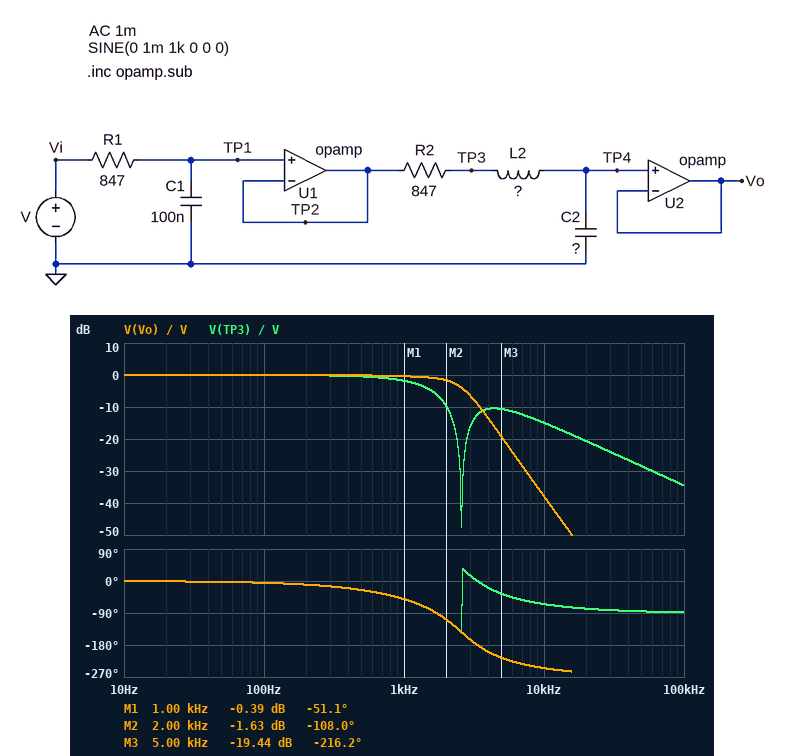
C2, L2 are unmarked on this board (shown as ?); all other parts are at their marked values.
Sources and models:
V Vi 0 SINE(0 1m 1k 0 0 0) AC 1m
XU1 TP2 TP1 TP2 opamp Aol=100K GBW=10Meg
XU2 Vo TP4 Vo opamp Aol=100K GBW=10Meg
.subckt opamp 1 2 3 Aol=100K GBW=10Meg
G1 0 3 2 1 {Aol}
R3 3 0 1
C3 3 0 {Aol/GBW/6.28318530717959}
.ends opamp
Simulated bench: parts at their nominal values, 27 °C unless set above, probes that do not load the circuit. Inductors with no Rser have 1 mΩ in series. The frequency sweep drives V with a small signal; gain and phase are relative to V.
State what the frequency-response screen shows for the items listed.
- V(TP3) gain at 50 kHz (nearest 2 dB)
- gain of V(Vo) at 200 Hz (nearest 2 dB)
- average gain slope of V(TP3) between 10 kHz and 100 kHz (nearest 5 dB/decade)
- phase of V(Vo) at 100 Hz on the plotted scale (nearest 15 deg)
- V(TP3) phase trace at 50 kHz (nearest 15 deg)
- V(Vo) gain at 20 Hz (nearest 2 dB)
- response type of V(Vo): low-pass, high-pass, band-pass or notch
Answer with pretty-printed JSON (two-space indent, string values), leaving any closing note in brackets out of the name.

{
  "V(TP3) gain at 50 kHz": "-28 dB",
  "gain of V(Vo) at 200 Hz": "0 dB",
  "average gain slope of V(TP3) between 10 kHz and 100 kHz": "-20 dB/decade",
  "phase of V(Vo) at 100 Hz on the plotted scale": "0 deg",
  "V(TP3) phase trace at 50 kHz": "-90 deg",
  "V(Vo) gain at 20 Hz": "0 dB",
  "response type of V(Vo): low-pass, high-pass, band-pass or notch": "low-pass"
}
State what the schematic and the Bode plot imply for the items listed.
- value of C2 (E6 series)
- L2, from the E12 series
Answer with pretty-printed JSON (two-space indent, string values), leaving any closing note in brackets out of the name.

{
  "value of C2": "68 nF",
  "L2, from the E12 series": "56 mH"
}
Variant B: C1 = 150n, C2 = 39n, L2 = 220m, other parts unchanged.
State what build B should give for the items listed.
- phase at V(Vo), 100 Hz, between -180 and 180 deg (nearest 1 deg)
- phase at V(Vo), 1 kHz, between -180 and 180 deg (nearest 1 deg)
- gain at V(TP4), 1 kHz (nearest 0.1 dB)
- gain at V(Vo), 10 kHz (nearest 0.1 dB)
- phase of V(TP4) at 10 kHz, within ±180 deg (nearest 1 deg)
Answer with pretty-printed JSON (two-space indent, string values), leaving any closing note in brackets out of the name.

{
  "phase at V(Vo), 100 Hz, between -180 and 180 deg": "-6 deg",
  "phase at V(Vo), 1 kHz, between -180 and 180 deg": "-56 deg",
  "gain at V(TP4), 1 kHz": "1.0 dB",
  "gain at V(Vo), 10 kHz": "-48.5 dB",
  "phase of V(TP4) at 10 kHz, within ±180 deg": "101 deg"
}
